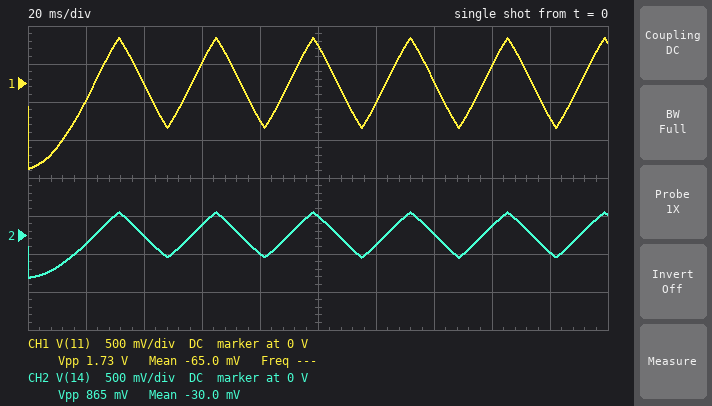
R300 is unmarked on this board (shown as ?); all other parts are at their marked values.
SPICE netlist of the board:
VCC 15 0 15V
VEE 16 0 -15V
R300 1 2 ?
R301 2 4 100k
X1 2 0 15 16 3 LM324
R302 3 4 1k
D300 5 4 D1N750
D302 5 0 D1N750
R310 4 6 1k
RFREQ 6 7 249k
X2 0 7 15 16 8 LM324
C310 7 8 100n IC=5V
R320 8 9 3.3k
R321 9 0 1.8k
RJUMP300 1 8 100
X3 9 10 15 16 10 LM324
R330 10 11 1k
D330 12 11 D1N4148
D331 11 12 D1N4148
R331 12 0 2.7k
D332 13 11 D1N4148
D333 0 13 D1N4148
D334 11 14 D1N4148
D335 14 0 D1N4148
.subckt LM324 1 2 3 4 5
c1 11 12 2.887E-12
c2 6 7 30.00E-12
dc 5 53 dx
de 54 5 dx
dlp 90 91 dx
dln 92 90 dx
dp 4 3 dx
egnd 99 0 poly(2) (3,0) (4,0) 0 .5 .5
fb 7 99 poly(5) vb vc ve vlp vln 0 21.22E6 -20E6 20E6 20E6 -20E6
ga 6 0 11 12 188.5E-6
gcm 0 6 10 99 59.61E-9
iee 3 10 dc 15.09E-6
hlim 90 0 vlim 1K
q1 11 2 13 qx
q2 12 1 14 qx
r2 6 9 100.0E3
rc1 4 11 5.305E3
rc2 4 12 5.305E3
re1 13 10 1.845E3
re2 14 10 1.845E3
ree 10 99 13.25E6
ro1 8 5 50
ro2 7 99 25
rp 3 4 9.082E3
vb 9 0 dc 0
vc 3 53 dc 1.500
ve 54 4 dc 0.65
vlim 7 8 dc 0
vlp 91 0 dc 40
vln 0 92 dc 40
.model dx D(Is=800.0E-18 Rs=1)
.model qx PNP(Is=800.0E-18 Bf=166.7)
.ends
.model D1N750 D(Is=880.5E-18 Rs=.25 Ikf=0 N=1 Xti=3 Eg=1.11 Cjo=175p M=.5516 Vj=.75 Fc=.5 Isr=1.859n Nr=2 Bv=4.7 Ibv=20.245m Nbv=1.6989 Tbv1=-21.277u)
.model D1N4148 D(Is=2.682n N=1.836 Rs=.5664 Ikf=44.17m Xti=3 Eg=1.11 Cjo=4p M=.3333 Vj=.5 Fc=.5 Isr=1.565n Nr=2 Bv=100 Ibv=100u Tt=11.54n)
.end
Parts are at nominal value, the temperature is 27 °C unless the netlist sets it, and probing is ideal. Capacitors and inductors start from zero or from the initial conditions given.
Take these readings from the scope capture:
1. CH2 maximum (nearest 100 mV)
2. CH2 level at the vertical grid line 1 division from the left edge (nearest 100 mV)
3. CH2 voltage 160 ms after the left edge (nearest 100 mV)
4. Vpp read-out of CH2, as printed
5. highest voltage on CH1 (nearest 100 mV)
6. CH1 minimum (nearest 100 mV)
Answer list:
300 mV
-100 mV
100 mV
865 mV
600 mV
-1.1 V
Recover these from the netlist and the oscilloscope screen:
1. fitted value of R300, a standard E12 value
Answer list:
33 kΩ
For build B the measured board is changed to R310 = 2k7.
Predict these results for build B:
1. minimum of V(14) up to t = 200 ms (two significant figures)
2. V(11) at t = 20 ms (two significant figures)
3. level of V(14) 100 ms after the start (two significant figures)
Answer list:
-570 mV
-240 mV
270 mV
